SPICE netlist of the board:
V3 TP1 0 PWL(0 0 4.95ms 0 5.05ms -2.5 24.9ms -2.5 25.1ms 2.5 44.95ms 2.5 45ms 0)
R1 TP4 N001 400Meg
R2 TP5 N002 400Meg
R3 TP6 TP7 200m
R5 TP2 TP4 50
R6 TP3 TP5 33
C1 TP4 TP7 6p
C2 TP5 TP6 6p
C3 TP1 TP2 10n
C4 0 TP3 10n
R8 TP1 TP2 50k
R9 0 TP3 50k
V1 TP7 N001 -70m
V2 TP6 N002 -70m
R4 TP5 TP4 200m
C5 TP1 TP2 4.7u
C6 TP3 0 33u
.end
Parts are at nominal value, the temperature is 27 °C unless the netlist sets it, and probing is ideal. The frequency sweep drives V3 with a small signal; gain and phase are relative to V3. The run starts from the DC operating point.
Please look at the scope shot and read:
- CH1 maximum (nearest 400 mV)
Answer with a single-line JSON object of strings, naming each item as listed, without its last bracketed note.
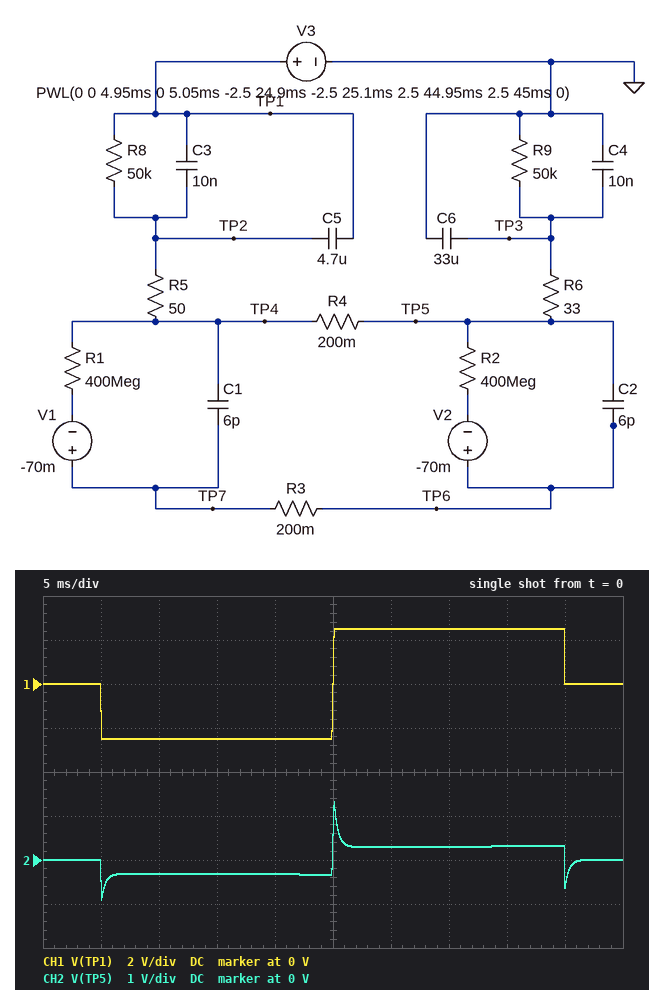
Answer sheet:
{"CH1 maximum": "2.4 V"}
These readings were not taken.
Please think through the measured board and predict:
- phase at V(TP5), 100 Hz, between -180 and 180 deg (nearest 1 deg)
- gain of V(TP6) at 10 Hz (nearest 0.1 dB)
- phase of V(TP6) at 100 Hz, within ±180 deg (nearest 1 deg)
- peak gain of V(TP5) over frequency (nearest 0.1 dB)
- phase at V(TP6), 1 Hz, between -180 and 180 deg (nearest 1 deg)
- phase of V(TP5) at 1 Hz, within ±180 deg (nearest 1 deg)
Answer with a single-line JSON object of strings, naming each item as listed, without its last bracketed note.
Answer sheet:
{"phase at V(TP5), 100 Hz, between -180 and 180 deg": "22 deg", "gain of V(TP6) at 10 Hz": "-18.0 dB", "phase of V(TP6) at 100 Hz, within ±180 deg": "22 deg", "peak gain of V(TP5) over frequency": "-6.0 dB", "phase at V(TP6), 1 Hz, between -180 and 180 deg": "-24 deg", "phase of V(TP5) at 1 Hz, within ±180 deg": "-24 deg"}
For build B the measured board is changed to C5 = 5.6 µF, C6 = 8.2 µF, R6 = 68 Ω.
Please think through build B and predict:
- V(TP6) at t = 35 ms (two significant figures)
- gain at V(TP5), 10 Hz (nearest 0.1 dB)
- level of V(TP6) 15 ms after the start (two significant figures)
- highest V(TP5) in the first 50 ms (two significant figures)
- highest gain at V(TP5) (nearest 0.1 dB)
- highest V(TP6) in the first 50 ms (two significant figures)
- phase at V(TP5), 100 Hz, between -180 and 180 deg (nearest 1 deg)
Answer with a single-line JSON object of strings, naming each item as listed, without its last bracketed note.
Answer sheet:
{"V(TP6) at t = 35 ms": "940 mV", "gain at V(TP5), 10 Hz": "-7.8 dB", "level of V(TP6) 15 ms after the start": "-1.1 V", "highest V(TP5) in the first 50 ms": "1.7 V", "highest gain at V(TP5)": "-4.8 dB", "highest V(TP6) in the first 50 ms": "1.6 V", "phase at V(TP5), 100 Hz, between -180 and 180 deg": "5 deg"}
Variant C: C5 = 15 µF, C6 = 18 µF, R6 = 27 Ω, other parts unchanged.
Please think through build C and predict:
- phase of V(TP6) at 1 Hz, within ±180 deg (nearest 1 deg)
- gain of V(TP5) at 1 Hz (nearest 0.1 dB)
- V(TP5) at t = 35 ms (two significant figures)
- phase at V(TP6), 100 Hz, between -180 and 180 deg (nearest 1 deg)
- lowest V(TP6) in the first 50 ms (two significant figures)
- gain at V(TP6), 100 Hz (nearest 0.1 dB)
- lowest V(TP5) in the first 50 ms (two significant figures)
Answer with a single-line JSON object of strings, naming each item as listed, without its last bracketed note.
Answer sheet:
{"phase of V(TP6) at 1 Hz, within ±180 deg": "-1 deg", "gain of V(TP5) at 1 Hz": "-6.8 dB", "V(TP5) at t = 35 ms": "1.1 V", "phase at V(TP6), 100 Hz, between -180 and 180 deg": "-5 deg", "lowest V(TP6) in the first 50 ms": "-1.2 V", "gain at V(TP6), 100 Hz": "-7.1 dB", "lowest V(TP5) in the first 50 ms": "-1.1 V"}
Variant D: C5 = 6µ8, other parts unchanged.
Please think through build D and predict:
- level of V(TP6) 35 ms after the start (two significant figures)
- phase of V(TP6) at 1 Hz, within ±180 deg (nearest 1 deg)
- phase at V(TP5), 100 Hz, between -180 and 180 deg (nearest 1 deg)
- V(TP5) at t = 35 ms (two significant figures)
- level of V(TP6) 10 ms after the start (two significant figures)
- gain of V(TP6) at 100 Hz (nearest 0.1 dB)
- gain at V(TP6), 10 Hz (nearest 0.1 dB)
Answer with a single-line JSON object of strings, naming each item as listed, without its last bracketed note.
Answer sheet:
{"level of V(TP6) 35 ms after the start": "350 mV", "phase of V(TP6) at 1 Hz, within ±180 deg": "-16 deg", "phase at V(TP5), 100 Hz, between -180 and 180 deg": "18 deg", "V(TP5) at t = 35 ms": "420 mV", "level of V(TP6) 10 ms after the start": "-500 mV", "gain of V(TP6) at 100 Hz": "-14.0 dB", "gain at V(TP6), 10 Hz": "-15.3 dB"}
